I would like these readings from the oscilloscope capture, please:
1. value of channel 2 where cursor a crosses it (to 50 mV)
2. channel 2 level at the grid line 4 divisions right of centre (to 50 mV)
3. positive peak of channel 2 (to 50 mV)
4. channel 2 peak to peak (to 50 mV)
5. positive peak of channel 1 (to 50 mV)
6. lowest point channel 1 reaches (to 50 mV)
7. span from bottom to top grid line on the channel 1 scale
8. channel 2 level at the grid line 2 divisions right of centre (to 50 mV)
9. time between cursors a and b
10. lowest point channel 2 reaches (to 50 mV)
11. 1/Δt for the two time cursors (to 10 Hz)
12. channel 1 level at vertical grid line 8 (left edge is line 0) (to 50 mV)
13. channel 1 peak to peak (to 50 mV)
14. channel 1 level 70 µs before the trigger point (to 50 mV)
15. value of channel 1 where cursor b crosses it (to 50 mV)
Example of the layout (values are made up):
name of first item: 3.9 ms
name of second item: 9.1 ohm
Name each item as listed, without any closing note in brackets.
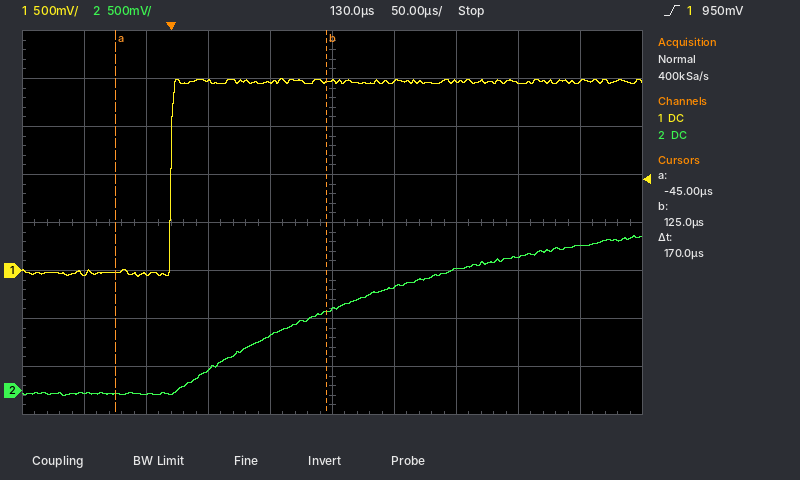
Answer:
value of channel 2 where cursor a crosses it: -50 mV
channel 2 level at the grid line 4 divisions right of centre: 1.50 V
positive peak of channel 2: 1.60 V
channel 2 peak to peak: 1.65 V
positive peak of channel 1: 2.00 V
lowest point channel 1 reaches: -50 mV
span from bottom to top grid line on the channel 1 scale: 4 V
channel 2 level at the grid line 2 divisions right of centre: 1.25 V
time between cursors a and b: 170 µs
lowest point channel 2 reaches: -50 mV
1/Δt for the two time cursors: 5.88 kHz
channel 1 level at vertical grid line 8 (left edge is line 0): 1.95 V
channel 1 peak to peak: 2.05 V
channel 1 level 70 µs before the trigger point: -50 mV
value of channel 1 where cursor b crosses it: 1.95 V
